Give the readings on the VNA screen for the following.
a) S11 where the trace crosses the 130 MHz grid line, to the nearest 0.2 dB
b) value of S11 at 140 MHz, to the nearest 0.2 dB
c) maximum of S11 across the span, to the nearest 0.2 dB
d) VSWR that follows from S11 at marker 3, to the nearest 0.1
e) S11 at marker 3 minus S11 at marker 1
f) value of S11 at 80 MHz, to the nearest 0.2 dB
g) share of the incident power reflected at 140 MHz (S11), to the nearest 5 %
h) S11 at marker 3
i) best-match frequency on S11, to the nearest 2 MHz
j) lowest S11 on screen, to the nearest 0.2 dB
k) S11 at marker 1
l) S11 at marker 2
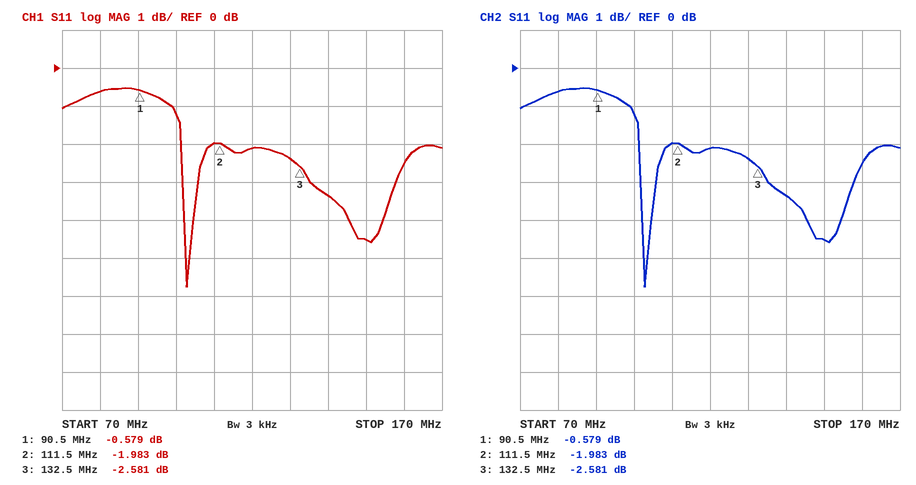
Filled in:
-2.4 dB
-3.4 dB
-0.6 dB
6.8
-2.002 dB
-0.6 dB
45 %
-2.581 dB
102 MHz
-5.8 dB
-0.579 dB
-1.983 dB
